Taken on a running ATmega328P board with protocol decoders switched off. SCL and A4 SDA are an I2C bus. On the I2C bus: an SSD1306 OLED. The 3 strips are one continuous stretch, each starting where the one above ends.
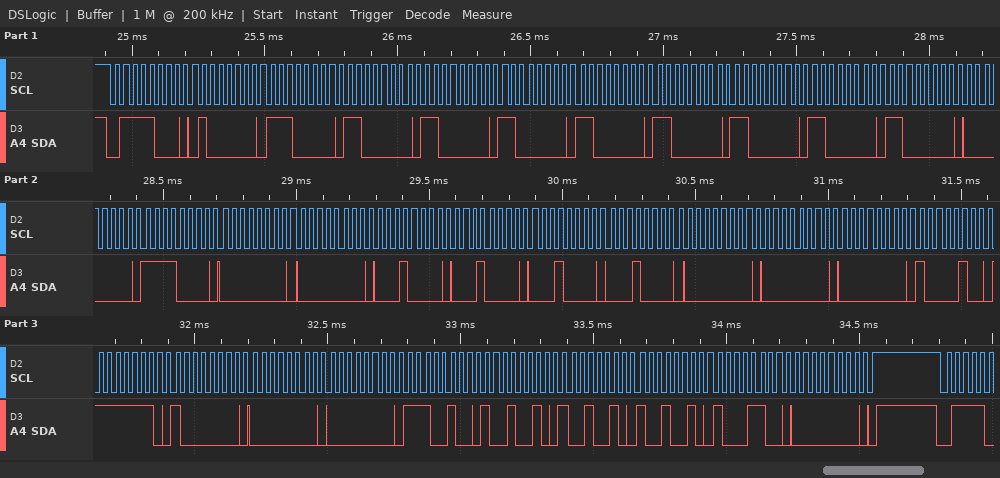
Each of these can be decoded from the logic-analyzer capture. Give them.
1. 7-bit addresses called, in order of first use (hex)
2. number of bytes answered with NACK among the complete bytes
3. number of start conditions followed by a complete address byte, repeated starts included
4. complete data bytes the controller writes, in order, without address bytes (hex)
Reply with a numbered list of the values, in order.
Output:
1. 0x3C
2. 0
3. 1
4. 40 E0 C0 C0 C0 C0 C0 C0 C0 C0 00 F0 00 00 10 10 10 10 00 00 00 84 FE 80 00 00 E4 92 92 92 8C 00
